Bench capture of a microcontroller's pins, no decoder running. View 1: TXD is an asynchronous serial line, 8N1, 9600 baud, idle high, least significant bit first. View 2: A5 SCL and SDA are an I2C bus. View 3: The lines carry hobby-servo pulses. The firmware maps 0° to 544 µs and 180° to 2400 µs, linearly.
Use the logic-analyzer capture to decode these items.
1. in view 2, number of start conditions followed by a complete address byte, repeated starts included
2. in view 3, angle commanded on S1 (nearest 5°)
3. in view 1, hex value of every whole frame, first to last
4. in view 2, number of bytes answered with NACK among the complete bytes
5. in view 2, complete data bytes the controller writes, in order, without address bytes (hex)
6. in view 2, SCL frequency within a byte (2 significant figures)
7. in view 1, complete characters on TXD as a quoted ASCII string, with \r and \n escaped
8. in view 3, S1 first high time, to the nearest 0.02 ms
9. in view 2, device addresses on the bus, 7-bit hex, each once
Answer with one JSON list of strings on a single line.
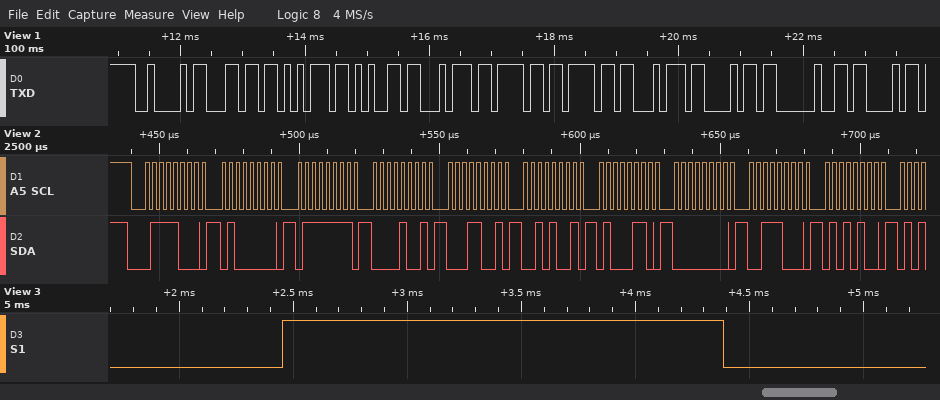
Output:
["1", "135°", "0x42 0x6C 0x75 0x65 0x74 0x6F 0x6F 0x74 0x68 0x20 0x43", "0", "40 7F 09 19 29 46 00 38 54", "400 kHz", "\"Bluetooth C\"", "1.94 ms", "0x3C"]
